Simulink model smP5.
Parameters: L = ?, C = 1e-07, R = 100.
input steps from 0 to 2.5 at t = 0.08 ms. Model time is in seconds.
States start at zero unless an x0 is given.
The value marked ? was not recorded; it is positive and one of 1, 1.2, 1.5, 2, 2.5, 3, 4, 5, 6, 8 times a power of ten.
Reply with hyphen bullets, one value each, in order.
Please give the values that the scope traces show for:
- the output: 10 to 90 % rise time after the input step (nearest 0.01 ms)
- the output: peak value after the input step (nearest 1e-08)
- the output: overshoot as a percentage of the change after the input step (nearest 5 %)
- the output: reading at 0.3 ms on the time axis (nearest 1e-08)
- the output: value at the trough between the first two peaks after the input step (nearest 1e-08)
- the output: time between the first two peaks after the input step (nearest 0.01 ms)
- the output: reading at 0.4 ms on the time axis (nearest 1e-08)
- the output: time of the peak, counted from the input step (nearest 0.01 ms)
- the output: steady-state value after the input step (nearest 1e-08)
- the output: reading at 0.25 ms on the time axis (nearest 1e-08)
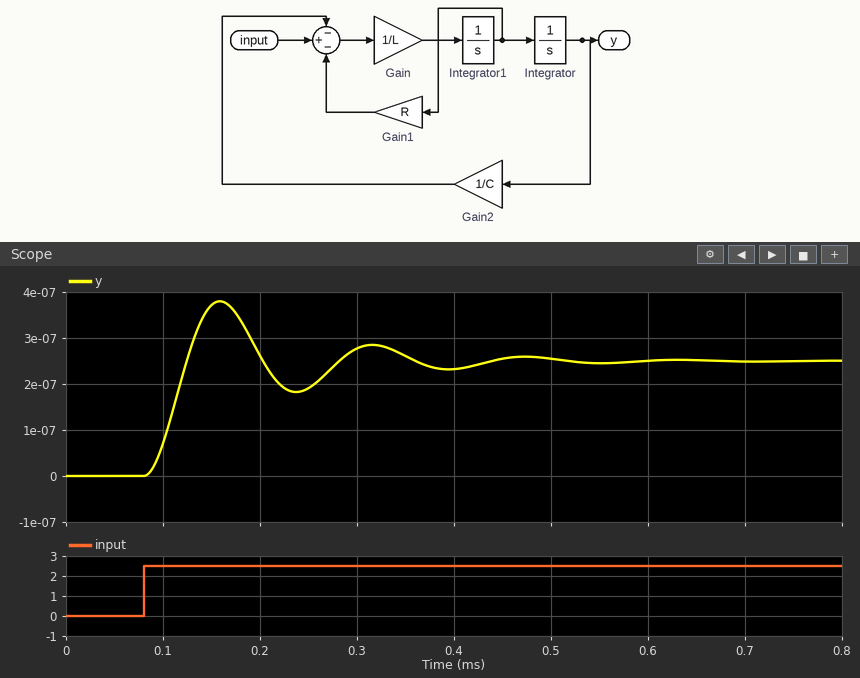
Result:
- 0.03 ms
- 0.00000038
- 50 %
- 0.00000028
- 0.00000018
- 0.16 ms
- 0.00000023
- 0.08 ms
- 0.00000025
- 0.00000019
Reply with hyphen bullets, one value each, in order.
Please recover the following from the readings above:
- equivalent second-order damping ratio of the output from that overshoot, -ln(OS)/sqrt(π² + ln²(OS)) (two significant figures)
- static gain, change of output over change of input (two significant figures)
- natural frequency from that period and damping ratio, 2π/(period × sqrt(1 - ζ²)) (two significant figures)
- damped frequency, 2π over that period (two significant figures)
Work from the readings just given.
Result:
- 0.22
- 0.00000010
- 40 rad/ms
- 39 rad/ms
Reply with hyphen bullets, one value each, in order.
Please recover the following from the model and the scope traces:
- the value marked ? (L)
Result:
- 0.006
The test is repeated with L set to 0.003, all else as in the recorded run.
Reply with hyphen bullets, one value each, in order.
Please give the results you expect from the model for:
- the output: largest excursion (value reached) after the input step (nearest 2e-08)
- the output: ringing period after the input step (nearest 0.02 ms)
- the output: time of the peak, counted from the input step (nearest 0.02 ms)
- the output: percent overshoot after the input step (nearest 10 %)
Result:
- 0.00000034
- 0.12 ms
- 0.06 ms
- 40 %
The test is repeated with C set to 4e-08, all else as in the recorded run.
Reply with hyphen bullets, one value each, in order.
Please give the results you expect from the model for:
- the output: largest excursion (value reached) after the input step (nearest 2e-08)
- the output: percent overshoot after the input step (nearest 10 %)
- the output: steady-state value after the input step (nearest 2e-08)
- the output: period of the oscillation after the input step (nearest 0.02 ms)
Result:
- 0.00000016
- 70 %
- 0.00000010
- 0.10 ms
